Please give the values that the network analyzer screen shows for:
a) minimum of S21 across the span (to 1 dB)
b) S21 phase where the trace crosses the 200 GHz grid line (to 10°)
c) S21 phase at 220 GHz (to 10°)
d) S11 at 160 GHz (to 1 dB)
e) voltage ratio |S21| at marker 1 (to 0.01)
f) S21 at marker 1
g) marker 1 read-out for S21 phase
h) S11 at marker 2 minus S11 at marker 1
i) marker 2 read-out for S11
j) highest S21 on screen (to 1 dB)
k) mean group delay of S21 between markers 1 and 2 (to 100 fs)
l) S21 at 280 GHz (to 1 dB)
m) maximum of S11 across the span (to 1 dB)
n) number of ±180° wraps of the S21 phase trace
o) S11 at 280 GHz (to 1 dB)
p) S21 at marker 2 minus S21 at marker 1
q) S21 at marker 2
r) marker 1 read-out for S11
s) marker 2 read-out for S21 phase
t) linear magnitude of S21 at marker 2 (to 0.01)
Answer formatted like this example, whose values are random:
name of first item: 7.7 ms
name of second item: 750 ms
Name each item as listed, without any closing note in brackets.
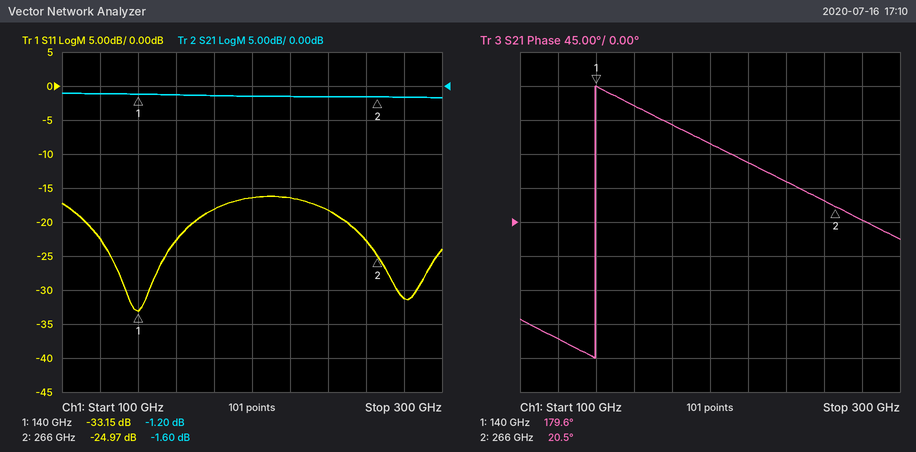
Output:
minimum of S21 across the span: -2 dB
S21 phase where the trace crosses the 200 GHz grid line: 100°
S21 phase at 220 GHz: 80°
S11 at 160 GHz: -23 dB
voltage ratio |S21| at marker 1: 0.87
S21 at marker 1: -1.20 dB
marker 1 read-out for S21 phase: 179.6°
S11 at marker 2 minus S11 at marker 1: 8.18 dB
marker 2 read-out for S11: -24.97 dB
highest S21 on screen: -1 dB
mean group delay of S21 between markers 1 and 2: 3.5 ps
S21 at 280 GHz: -2 dB
maximum of S11 across the span: -16 dB
number of ±180° wraps of the S21 phase trace: 1
S11 at 280 GHz: -31 dB
S21 at marker 2 minus S21 at marker 1: -0.40 dB
S21 at marker 2: -1.60 dB
marker 1 read-out for S11: -33.15 dB
marker 2 read-out for S21 phase: 20.5°
linear magnitude of S21 at marker 2: 0.83
